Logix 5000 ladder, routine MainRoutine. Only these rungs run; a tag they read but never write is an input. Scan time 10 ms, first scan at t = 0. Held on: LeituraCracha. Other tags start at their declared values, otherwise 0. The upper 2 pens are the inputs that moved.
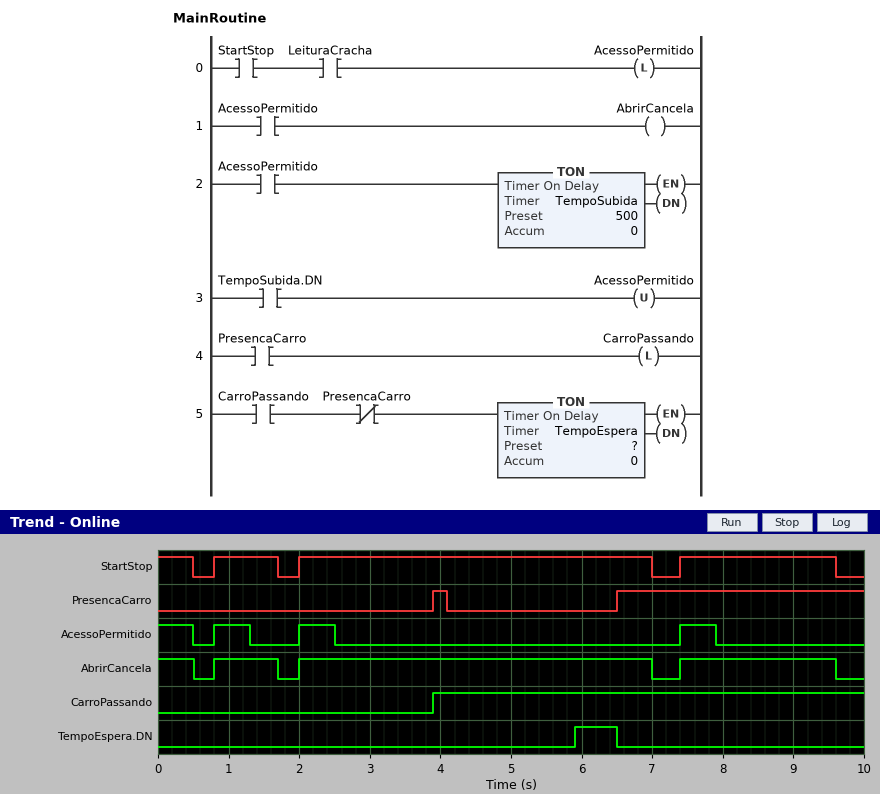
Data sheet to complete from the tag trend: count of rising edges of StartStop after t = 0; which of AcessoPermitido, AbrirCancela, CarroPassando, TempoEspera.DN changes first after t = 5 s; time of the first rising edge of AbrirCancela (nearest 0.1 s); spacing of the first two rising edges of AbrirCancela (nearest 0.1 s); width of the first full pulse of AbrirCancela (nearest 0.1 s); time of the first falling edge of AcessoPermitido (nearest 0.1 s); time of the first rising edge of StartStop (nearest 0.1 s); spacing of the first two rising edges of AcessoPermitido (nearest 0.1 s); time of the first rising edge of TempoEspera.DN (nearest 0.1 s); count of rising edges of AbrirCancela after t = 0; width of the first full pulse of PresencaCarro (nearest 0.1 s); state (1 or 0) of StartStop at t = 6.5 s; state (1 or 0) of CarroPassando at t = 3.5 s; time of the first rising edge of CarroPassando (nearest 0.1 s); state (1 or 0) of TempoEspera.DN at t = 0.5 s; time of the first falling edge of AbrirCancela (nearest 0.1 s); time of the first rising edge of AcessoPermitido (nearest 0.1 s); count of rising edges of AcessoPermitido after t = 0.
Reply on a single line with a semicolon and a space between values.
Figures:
3; TempoEspera.DN; 0.8 s; 1.2 s; 0.9 s; 0.5 s; 0.8 s; 1.2 s; 5.9 s; 3; 0.2 s; 1; 0; 3.9 s; 0; 0.5 s; 0.8 s; 3
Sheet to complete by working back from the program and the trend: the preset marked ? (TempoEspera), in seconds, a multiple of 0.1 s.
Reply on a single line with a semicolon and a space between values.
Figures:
1.8 s
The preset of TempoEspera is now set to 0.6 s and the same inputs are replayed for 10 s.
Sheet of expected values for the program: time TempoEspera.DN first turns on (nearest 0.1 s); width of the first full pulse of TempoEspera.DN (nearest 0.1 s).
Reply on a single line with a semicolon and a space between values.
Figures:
4.7 s; 1.8 s
